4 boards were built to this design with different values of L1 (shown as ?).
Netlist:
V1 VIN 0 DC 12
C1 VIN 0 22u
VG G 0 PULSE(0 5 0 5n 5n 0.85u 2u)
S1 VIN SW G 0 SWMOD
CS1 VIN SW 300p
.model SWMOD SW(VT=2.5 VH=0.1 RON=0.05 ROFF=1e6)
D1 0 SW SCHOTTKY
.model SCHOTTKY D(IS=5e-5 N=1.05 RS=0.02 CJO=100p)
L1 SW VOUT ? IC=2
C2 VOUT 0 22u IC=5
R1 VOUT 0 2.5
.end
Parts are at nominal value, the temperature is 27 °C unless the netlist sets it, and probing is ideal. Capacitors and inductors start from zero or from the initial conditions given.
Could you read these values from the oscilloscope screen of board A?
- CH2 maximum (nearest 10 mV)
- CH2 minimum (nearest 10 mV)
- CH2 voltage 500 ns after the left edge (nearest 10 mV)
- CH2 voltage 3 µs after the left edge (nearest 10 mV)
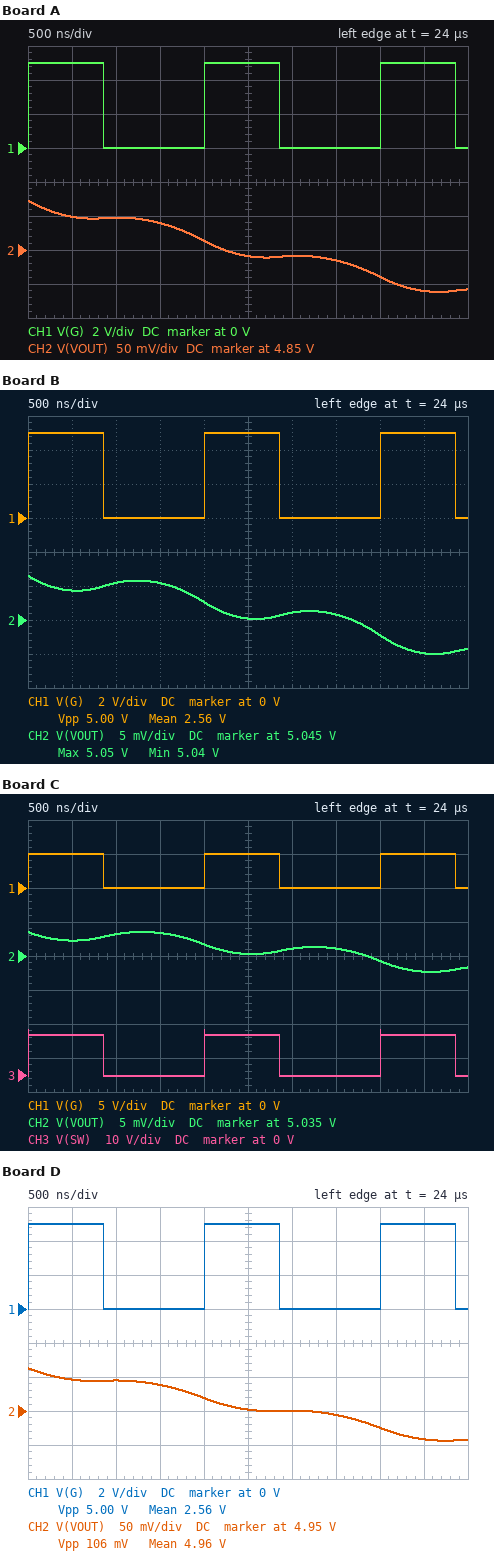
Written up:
4.92 V
4.79 V
4.90 V
4.84 V
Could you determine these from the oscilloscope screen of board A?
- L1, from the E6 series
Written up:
3.3 µH
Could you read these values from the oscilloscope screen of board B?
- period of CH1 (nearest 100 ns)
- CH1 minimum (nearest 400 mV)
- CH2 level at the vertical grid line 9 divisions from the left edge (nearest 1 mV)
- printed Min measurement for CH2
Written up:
2.0 µs
0 V
5.040 V
5.04 V
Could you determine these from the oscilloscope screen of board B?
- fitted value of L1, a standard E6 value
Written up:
22 µH
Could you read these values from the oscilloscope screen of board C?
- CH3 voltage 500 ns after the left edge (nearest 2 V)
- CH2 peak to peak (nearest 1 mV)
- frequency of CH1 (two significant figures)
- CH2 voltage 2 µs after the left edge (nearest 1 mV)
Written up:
12 V
6 mV
500 kHz
5.037 V
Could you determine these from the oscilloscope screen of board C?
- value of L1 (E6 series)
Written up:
33 µH
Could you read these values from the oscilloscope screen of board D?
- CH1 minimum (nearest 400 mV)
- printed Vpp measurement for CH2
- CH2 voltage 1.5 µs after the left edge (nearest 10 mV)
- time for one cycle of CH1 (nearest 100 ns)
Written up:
0 V
106 mV
4.99 V
2.0 µs
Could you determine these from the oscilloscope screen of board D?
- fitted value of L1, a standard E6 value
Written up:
4.7 µH
